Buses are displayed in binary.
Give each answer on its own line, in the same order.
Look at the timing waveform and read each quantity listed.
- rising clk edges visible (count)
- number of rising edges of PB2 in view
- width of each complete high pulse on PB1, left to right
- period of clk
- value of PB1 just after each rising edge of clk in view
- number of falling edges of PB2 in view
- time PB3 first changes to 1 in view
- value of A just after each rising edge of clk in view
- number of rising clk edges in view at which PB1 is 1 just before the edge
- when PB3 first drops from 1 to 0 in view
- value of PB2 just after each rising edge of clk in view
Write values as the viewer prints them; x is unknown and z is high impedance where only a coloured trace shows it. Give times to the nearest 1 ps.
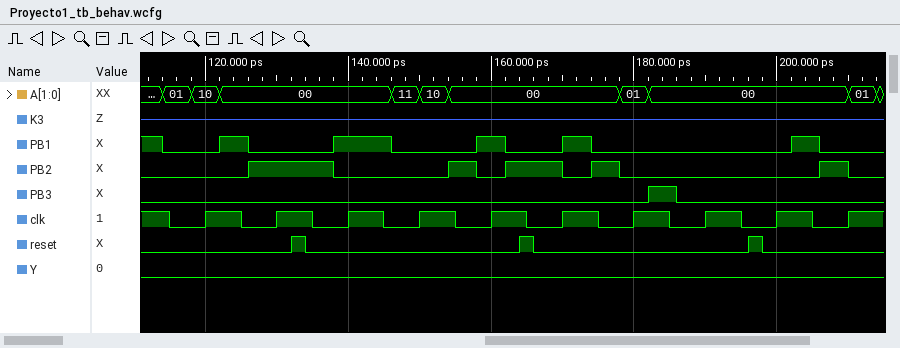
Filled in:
10
5
4 ps, 8 ps, 4 ps, 4 ps, 4 ps
10 ps
0 0 1 0 1 1 0 0 0 0
5
182 ps
10, 00, 00, 10, 00, 00, 01, 00, 00, 01
2
186 ps
0 1 0 0 0 0 0 0 0 0
